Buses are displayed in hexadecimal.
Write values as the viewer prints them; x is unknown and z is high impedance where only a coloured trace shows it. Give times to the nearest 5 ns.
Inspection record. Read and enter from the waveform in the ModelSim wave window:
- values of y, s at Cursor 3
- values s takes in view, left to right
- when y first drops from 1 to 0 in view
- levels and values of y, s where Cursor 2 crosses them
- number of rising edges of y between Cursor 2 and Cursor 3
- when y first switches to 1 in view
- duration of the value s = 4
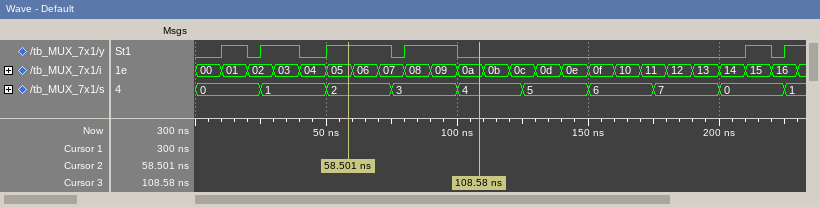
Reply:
y=0, s=4
0, 1, 2, 3, 4, 5, 6, 7, 0, 1
20 ns
y=1, s=2
1
10 ns
25 ns
